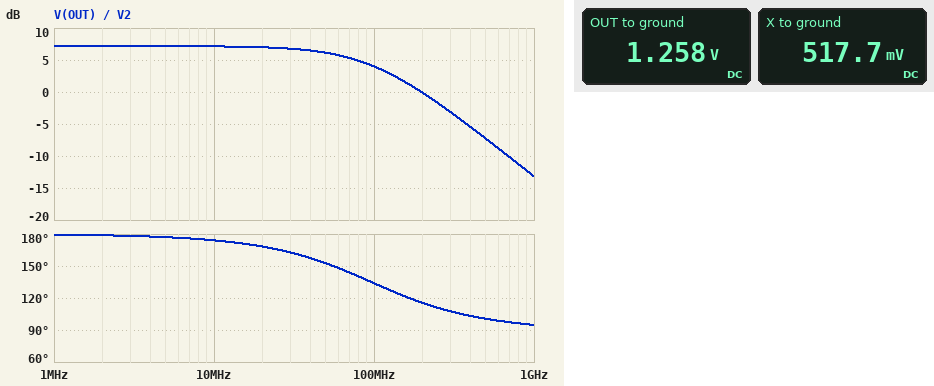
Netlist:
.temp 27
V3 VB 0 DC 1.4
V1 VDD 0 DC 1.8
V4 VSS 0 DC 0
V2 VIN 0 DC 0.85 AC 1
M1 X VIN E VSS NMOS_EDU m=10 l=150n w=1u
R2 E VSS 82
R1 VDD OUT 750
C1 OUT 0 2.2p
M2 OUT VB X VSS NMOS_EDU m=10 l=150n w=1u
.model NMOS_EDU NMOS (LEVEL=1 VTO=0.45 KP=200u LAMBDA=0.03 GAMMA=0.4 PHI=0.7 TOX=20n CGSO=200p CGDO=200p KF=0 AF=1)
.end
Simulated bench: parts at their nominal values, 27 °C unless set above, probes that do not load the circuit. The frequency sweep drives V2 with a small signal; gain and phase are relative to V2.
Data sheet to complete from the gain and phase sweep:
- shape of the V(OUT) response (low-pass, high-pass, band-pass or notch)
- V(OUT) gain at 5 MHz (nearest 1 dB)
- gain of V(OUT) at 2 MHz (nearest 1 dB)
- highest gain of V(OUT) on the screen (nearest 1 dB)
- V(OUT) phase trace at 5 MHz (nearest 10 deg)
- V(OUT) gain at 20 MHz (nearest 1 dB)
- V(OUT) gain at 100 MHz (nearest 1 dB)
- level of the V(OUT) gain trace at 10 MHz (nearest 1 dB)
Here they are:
low-pass
7 dB
7 dB
7 dB
180 deg
7 dB
4 dB
7 dB
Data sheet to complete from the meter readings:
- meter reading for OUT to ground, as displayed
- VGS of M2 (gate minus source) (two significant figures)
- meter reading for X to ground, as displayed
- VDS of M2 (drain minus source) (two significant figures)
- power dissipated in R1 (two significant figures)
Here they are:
1.258 V
880 mV
517.7 mV
740 mV
390 µW
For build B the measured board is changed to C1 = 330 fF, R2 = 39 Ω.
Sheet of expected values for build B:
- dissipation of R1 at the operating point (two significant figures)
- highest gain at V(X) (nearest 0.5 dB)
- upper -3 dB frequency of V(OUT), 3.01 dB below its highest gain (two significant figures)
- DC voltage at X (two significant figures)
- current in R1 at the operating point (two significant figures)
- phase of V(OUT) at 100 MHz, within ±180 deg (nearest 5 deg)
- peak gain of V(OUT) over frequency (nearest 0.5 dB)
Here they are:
560 µW
-3.0 dB
640 MHz
490 mV
870 µA
170 deg
9.5 dB
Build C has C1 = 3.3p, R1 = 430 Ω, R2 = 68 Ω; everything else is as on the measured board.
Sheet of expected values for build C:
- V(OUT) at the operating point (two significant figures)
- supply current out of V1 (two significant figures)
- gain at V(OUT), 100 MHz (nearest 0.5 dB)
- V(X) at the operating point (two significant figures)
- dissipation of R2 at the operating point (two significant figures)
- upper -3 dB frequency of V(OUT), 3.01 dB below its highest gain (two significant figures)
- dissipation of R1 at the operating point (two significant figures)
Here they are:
1.5 V
760 µA
0.5 dB
510 mV
40 µW
110 MHz
250 µW
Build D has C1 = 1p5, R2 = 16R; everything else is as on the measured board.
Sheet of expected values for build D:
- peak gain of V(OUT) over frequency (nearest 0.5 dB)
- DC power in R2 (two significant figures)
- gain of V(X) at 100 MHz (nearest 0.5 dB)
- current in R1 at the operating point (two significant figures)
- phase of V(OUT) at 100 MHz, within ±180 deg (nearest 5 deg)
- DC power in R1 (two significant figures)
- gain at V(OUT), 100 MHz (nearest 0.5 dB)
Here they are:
11.0 dB
15 µW
-2.5 dB
980 µA
145 deg
720 µW
9.0 dB
